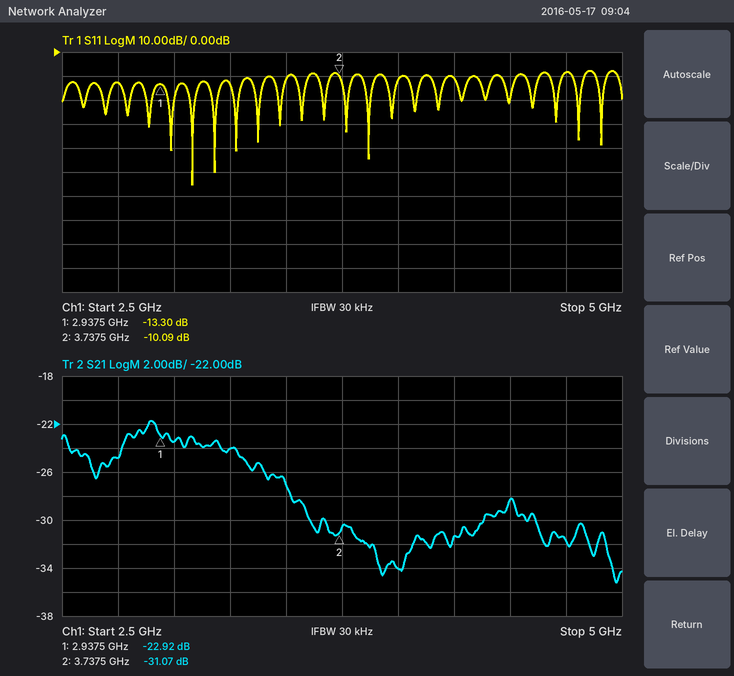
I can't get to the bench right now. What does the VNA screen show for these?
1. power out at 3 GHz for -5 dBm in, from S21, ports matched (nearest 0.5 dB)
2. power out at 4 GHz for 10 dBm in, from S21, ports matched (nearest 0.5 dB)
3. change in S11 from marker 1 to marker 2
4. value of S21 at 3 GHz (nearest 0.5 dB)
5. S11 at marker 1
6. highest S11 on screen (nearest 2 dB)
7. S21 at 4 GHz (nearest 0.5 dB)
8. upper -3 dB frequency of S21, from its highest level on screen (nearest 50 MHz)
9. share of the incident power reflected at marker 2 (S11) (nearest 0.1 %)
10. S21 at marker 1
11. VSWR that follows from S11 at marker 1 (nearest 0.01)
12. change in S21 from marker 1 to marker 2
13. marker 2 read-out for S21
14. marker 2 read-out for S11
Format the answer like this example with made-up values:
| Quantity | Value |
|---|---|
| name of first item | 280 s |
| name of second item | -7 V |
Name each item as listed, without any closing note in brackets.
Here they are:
| Quantity | Value |
|---|---|
| power out at 3 GHz for -5 dBm in, from S21, ports matched | -28.5 dBm |
| power out at 4 GHz for 10 dBm in, from S21, ports matched | -24.0 dBm |
| change in S11 from marker 1 to marker 2 | 3.21 dB |
| value of S21 at 3 GHz | -23.5 dB |
| S11 at marker 1 | -13.30 dB |
| highest S11 on screen | -8 dB |
| S21 at 4 GHz | -34.0 dB |
| upper -3 dB frequency of S21, from its highest level on screen | 3.30 GHz |
| share of the incident power reflected at marker 2 (S11) | 9.8 % |
| S21 at marker 1 | -22.92 dB |
| VSWR that follows from S11 at marker 1 | 1.55 |
| change in S21 from marker 1 to marker 2 | -8.15 dB |
| marker 2 read-out for S21 | -31.07 dB |
| marker 2 read-out for S11 | -10.09 dB |
